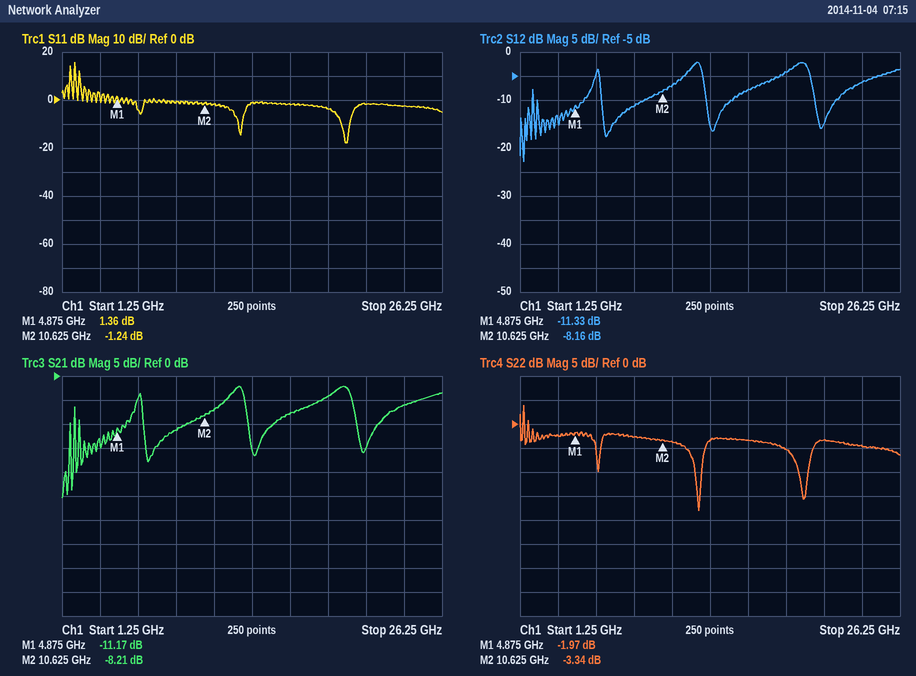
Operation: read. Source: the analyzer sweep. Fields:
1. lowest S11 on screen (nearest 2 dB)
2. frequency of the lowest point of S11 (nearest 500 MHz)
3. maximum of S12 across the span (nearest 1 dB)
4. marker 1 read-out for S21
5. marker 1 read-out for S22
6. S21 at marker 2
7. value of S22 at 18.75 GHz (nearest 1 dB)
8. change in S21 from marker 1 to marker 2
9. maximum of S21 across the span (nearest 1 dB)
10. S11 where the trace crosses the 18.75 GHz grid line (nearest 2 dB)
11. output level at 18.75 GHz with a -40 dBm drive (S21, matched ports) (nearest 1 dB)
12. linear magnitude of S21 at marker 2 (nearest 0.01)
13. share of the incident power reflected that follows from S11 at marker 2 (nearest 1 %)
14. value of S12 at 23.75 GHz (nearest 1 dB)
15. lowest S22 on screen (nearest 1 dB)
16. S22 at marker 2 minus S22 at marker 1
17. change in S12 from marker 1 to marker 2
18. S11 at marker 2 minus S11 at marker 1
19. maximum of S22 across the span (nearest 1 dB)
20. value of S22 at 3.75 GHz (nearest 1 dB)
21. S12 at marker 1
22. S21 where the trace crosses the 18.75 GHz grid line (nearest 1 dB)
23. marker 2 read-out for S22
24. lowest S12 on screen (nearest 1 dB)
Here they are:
-18 dB
20.0 GHz
-2 dB
-11.17 dB
-1.97 dB
-8.21 dB
-5 dB
2.96 dB
-2 dB
-4 dB
-44 dBm
0.39
75 %
-6 dB
-18 dB
-1.37 dB
3.17 dB
-2.60 dB
4 dB
-2 dB
-11.33 dB
-4 dB
-3.34 dB
-23 dB
